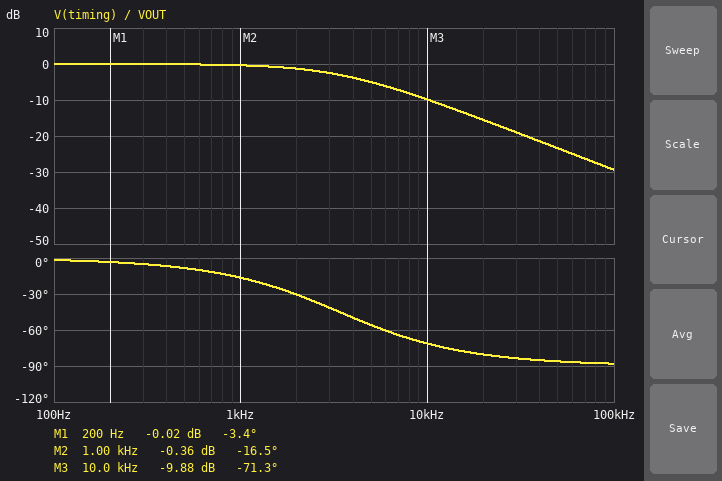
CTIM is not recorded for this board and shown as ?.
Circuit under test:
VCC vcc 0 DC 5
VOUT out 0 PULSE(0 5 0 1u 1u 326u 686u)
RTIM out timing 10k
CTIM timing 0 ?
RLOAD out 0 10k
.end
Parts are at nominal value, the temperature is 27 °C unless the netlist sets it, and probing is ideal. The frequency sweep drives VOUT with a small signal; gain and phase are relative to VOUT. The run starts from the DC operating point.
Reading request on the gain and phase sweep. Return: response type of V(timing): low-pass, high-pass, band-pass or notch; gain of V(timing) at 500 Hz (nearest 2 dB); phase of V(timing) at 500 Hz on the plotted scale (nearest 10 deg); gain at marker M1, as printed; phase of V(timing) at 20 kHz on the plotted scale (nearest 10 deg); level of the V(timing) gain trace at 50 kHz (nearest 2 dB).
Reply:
low-pass
0 dB
-10 deg
-0.02 dB
-80 deg
-24 dB
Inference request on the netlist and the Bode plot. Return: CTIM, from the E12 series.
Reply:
4.7 nF
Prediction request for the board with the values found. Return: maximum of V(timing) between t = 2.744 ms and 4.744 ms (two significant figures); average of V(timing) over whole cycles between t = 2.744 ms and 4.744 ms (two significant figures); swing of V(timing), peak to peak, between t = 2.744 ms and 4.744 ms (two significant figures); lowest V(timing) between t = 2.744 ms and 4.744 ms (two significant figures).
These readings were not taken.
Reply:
5.0 V
2.4 V
5.0 V
2.4 mV
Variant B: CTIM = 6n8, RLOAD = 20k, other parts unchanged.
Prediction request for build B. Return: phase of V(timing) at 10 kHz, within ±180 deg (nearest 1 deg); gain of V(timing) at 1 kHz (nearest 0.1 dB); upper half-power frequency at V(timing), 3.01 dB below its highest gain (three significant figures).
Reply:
-77 deg
-0.7 dB
2.34 kHz
